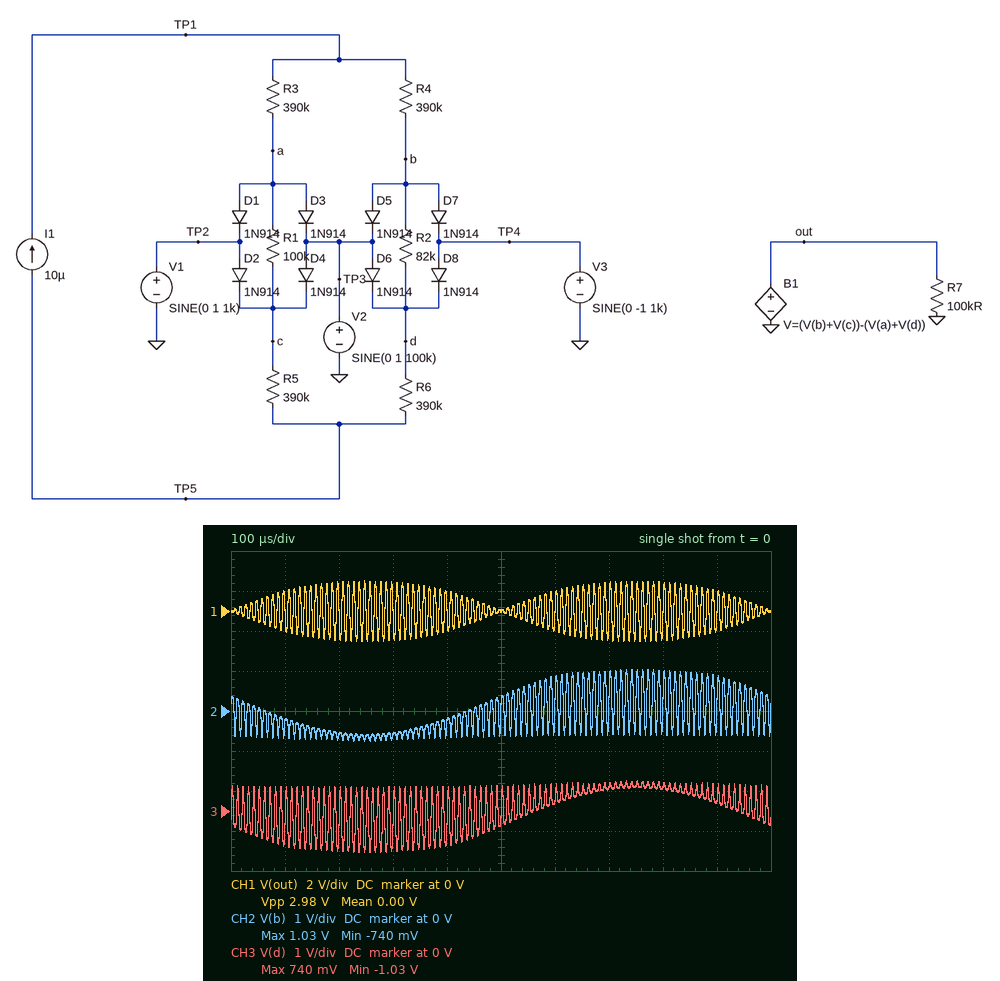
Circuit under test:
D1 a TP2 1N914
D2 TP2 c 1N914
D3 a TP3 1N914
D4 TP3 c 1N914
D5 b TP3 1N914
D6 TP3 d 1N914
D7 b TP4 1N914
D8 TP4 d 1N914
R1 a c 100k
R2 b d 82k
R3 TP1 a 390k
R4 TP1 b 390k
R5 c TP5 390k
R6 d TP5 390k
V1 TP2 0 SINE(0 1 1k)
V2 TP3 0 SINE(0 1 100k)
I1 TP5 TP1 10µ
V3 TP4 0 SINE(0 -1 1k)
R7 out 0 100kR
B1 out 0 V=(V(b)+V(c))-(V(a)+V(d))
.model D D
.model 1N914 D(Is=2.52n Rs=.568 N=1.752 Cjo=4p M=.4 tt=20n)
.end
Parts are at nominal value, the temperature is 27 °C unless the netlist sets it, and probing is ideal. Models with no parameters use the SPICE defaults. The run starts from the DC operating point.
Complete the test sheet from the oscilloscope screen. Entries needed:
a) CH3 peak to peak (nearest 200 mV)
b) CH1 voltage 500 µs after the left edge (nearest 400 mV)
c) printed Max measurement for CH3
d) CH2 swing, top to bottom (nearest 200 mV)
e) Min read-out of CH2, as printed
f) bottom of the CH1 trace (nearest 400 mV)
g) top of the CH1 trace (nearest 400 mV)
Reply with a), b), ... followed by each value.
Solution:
a) 1.8 V
b) 0 V
c) 740 mV
d) 1.8 V
e) -740 mV
f) -1.6 V
g) 1.6 V
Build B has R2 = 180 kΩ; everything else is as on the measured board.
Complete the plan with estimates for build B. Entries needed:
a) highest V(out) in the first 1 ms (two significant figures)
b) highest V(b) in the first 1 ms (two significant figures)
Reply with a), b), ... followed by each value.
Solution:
a) 1.6 V
b) 1.2 V
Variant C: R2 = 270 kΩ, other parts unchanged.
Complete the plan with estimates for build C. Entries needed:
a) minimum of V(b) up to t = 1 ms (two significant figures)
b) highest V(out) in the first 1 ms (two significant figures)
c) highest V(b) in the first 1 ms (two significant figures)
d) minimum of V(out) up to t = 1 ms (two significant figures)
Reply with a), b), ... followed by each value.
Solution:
a) -710 mV
b) 1.7 V
c) 1.2 V
d) -1.6 V
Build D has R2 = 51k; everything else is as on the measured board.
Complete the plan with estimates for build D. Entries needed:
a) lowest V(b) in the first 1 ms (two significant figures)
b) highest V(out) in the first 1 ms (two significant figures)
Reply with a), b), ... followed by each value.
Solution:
a) -760 mV
b) 1.4 V
